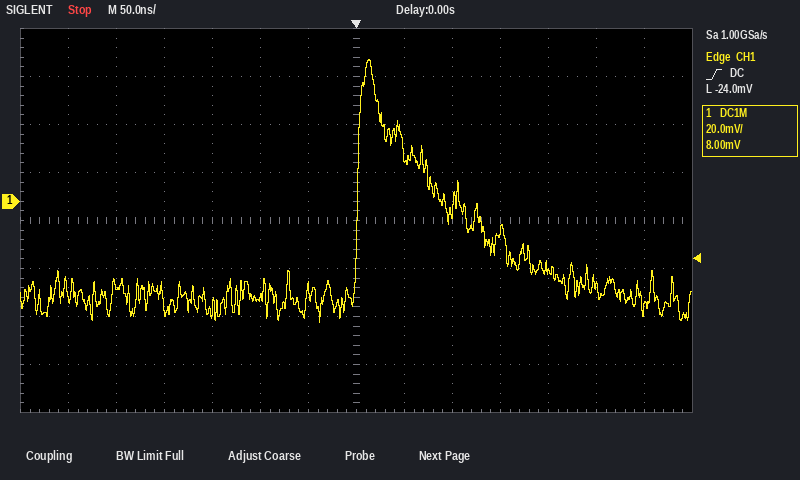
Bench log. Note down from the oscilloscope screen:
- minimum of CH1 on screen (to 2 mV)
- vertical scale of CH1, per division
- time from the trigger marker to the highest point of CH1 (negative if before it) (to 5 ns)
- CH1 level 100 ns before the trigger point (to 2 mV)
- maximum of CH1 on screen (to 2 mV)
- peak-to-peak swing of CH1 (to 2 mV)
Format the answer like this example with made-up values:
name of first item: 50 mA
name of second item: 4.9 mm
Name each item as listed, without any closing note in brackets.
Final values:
minimum of CH1 on screen: -50 mV
vertical scale of CH1, per division: 20 mV
time from the trigger marker to the highest point of CH1 (negative if before it): +15 ns
CH1 level 100 ns before the trigger point: -40 mV
maximum of CH1 on screen: 60 mV
peak-to-peak swing of CH1: 110 mV
